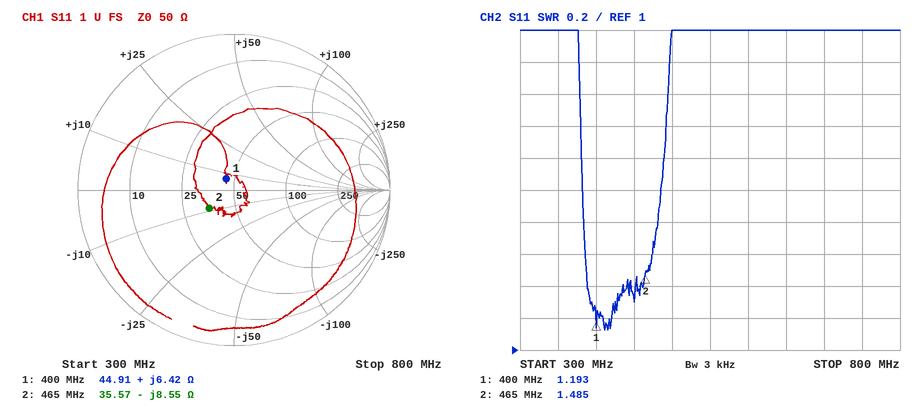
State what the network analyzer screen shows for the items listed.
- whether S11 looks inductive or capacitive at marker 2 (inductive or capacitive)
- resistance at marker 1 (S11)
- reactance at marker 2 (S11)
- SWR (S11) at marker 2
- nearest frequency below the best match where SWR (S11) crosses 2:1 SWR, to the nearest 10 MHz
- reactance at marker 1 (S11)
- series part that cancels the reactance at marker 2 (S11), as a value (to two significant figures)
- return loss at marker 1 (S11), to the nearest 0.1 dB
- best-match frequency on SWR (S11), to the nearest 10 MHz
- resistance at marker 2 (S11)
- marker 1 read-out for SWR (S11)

capacitive
44.91 Ω
-8.55 Ω
1.485
380 MHz
+6.42 Ω
2.9 nH
21.3 dB
410 MHz
35.57 Ω
1.193
